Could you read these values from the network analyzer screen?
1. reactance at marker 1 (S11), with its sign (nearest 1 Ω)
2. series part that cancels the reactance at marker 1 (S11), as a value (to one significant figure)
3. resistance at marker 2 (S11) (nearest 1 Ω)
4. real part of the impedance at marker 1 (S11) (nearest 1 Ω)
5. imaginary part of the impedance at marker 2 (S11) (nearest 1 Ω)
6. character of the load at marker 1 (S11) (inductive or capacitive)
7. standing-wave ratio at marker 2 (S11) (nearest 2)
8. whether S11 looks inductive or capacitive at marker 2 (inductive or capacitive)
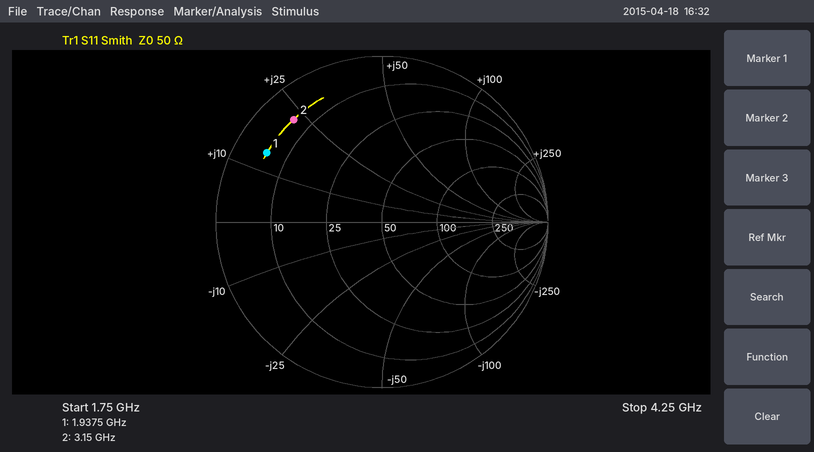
+14 Ω
6 pF
6 Ω
6 Ω
+23 Ω
inductive
10
inductive
